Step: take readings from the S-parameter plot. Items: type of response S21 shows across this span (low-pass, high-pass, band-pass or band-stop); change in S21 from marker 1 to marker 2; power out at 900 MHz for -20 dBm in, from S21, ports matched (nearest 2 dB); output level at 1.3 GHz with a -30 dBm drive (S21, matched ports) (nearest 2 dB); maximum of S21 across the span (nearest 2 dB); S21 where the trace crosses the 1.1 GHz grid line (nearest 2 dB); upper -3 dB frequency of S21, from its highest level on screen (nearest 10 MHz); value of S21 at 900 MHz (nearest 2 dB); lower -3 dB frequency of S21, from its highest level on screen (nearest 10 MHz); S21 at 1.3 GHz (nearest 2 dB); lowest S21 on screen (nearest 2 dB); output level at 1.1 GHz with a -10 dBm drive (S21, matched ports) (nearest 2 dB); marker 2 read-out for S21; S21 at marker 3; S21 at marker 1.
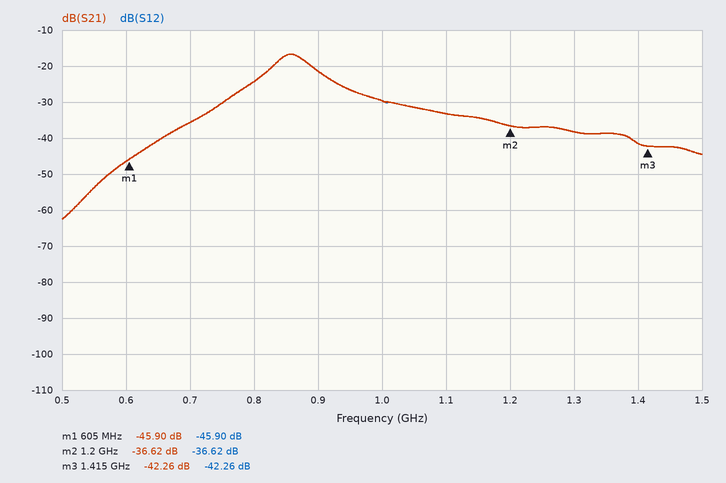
band-pass
9.28 dB
-42 dBm
-68 dBm
-16 dB
-34 dB
890 MHz
-22 dB
830 MHz
-38 dB
-62 dB
-44 dBm
-36.62 dB
-42.26 dB
-45.90 dB
